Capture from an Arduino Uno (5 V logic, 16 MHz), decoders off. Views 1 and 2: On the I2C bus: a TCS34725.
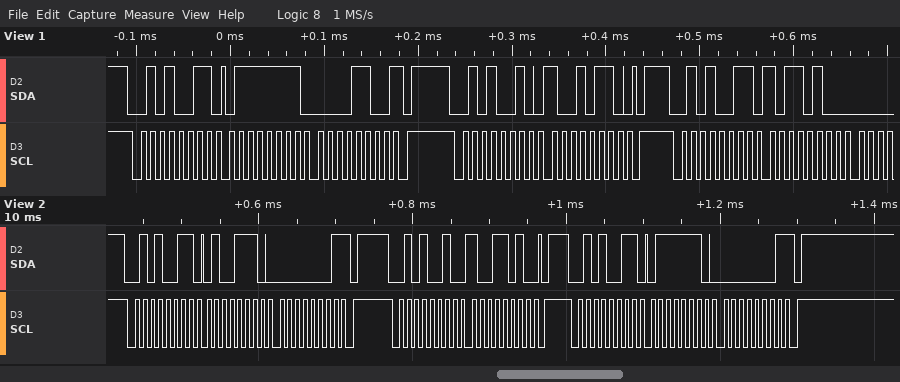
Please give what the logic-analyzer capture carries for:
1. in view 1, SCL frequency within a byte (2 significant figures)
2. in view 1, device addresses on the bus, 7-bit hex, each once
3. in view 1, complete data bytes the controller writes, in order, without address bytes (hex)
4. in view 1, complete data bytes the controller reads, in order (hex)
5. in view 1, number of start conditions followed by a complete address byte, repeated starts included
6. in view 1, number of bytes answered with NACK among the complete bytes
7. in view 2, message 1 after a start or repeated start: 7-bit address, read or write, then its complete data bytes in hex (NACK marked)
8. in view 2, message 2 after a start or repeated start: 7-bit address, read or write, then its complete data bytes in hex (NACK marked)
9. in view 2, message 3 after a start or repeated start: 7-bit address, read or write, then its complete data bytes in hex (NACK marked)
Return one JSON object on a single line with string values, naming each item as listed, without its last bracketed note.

{"in view 1, SCL frequency within a byte": "100 kHz", "in view 1, device addresses on the bus, 7-bit hex, each once": "0x29", "in view 1, complete data bytes the controller writes, in order, without address bytes": "96", "in view 1, complete data bytes the controller reads, in order": "7F 0C B4", "in view 1, number of start conditions followed by a complete address byte, repeated starts included": "3", "in view 1, number of bytes answered with NACK among the complete bytes": "1", "in view 2, message 1 after a start or repeated start: 7-bit address, read or write, then its complete data bytes in hex": "0x29 read: 4E 01 NACK", "in view 2, message 2 after a start or repeated start: 7-bit address, read or write, then its complete data bytes in hex": "0x29 write: 9A", "in view 2, message 3 after a start or repeated start: 7-bit address, read or write, then its complete data bytes in hex": "0x29 read: 7E 01 NACK"}
